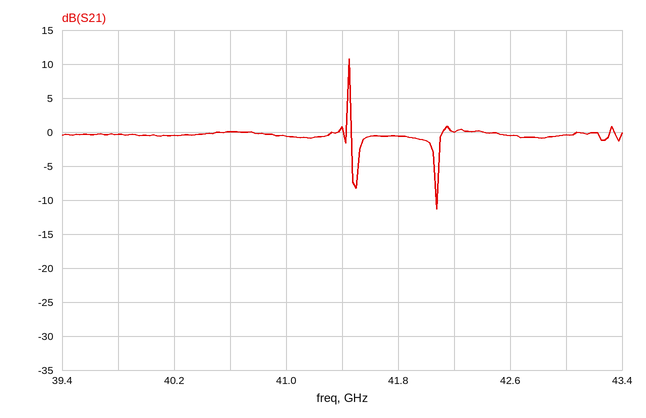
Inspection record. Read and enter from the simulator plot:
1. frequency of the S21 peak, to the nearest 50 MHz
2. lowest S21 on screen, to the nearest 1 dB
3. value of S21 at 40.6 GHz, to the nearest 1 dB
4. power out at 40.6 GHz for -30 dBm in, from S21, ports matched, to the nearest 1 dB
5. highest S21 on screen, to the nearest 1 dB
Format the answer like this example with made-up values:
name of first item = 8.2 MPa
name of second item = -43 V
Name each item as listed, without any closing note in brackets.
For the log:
frequency of the S21 peak, to the nearest 50 MHz = 41.45 GHz
lowest S21 on screen, to the nearest 1 dB = -11 dB
value of S21 at 40.6 GHz, to the nearest 1 dB = 0 dB
power out at 40.6 GHz for -30 dBm in, from S21, ports matched, to the nearest 1 dB = -30 dBm
highest S21 on screen, to the nearest 1 dB = 11 dB
